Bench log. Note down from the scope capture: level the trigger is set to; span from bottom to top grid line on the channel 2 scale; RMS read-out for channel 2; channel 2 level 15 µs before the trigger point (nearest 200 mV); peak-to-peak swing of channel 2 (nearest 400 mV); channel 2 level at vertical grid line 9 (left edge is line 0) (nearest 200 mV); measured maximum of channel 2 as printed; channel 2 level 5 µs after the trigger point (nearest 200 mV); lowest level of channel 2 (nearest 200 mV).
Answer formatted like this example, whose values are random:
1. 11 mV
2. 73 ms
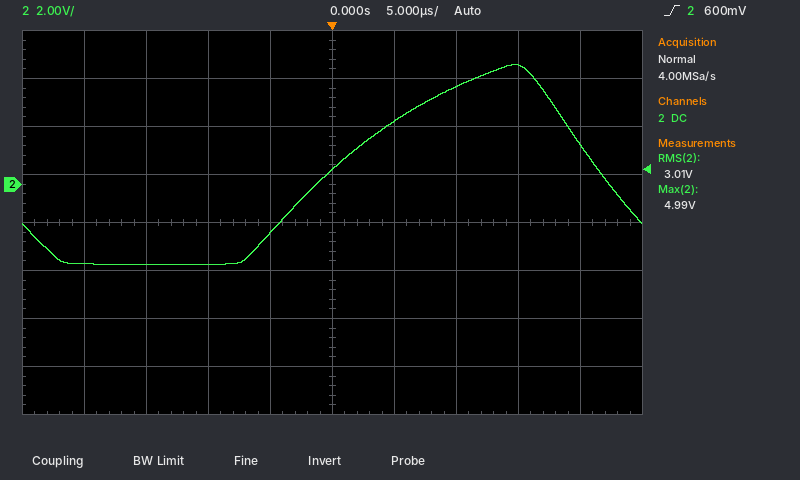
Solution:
1. 600 mV
2. 16 V
3. 3.01 V
4. -3.4 V
5. 8.4 V
6. 1.6 V
7. 4.99 V
8. 2.6 V
9. -3.4 V
